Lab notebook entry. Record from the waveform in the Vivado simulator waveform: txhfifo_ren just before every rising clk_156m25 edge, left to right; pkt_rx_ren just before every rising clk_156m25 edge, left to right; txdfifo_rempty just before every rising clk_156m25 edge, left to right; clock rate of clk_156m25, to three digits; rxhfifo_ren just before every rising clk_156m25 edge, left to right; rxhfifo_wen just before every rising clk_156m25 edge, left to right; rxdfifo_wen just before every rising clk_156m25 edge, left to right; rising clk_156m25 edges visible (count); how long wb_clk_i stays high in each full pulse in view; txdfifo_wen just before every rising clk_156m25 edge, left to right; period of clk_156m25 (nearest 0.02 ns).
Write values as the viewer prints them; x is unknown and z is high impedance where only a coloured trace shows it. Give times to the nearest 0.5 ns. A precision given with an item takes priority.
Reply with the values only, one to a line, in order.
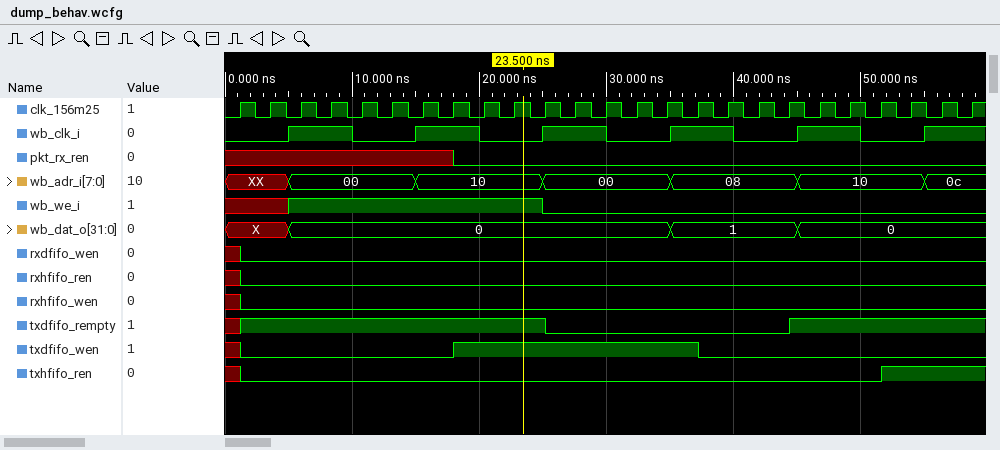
x 0 0 0 0 0 0 0 0 0 0 0 0 0 0 0 0 0 0 0 0 0 1 1 1
x x x x x x x x 0 0 0 0 0 0 0 0 0 0 0 0 0 0 0 0 0
x 1 1 1 1 1 1 1 1 1 1 0 0 0 0 0 0 0 0 1 1 1 1 1 1
417 MHz
x 0 0 0 0 0 0 0 0 0 0 0 0 0 0 0 0 0 0 0 0 0 0 0 0
x 0 0 0 0 0 0 0 0 0 0 0 0 0 0 0 0 0 0 0 0 0 0 0 0
x 0 0 0 0 0 0 0 0 0 0 0 0 0 0 0 0 0 0 0 0 0 0 0 0
25
5 ns, 5 ns, 5 ns, 5 ns, 5 ns
x 0 0 0 0 0 0 0 1 1 1 1 1 1 1 1 0 0 0 0 0 0 0 0 0
2.4 ns
